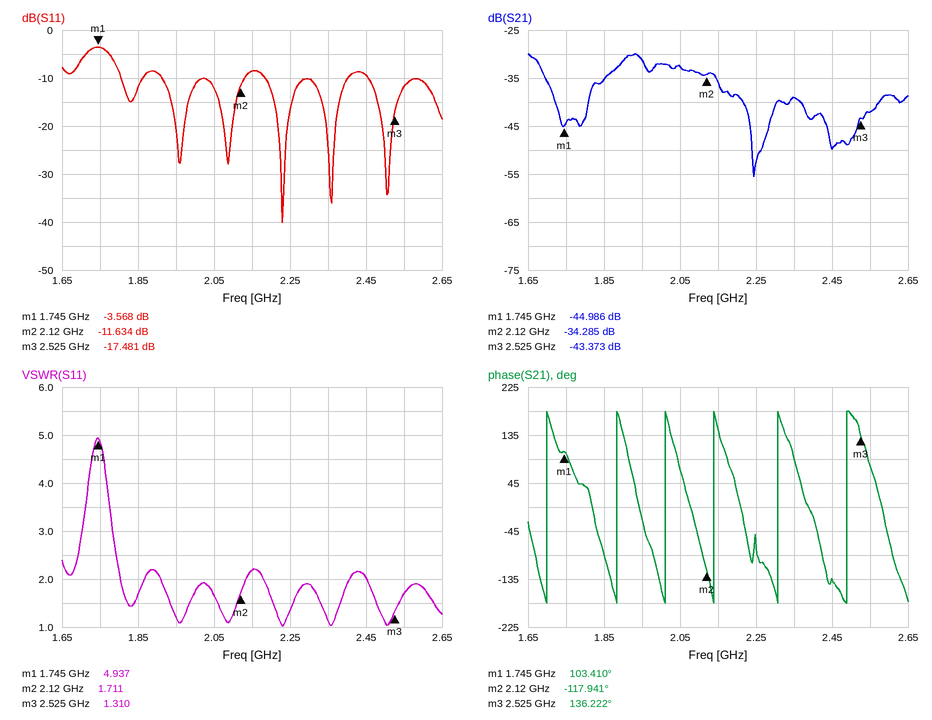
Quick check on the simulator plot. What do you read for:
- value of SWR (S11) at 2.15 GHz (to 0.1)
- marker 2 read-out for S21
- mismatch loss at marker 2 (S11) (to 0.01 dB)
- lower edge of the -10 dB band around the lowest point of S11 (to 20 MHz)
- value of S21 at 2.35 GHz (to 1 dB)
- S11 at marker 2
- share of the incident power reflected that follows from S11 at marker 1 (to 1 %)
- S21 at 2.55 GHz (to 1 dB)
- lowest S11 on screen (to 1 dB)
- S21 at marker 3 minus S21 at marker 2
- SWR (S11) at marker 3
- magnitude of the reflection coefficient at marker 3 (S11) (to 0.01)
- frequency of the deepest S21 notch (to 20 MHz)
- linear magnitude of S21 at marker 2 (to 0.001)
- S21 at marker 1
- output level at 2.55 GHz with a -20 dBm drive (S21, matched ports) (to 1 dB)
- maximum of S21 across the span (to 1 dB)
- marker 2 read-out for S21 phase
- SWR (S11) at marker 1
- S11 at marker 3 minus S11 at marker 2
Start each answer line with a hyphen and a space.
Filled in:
- 2.2
- -34.285 dB
- 0.31 dB
- 2.18 GHz
- -39 dB
- -11.634 dB
- 44 %
- -42 dB
- -40 dB
- -9.088 dB
- 1.310
- 0.13
- 2.24 GHz
- 0.019
- -44.986 dB
- -62 dBm
- -30 dB
- -117.941°
- 4.937
- -5.847 dB
